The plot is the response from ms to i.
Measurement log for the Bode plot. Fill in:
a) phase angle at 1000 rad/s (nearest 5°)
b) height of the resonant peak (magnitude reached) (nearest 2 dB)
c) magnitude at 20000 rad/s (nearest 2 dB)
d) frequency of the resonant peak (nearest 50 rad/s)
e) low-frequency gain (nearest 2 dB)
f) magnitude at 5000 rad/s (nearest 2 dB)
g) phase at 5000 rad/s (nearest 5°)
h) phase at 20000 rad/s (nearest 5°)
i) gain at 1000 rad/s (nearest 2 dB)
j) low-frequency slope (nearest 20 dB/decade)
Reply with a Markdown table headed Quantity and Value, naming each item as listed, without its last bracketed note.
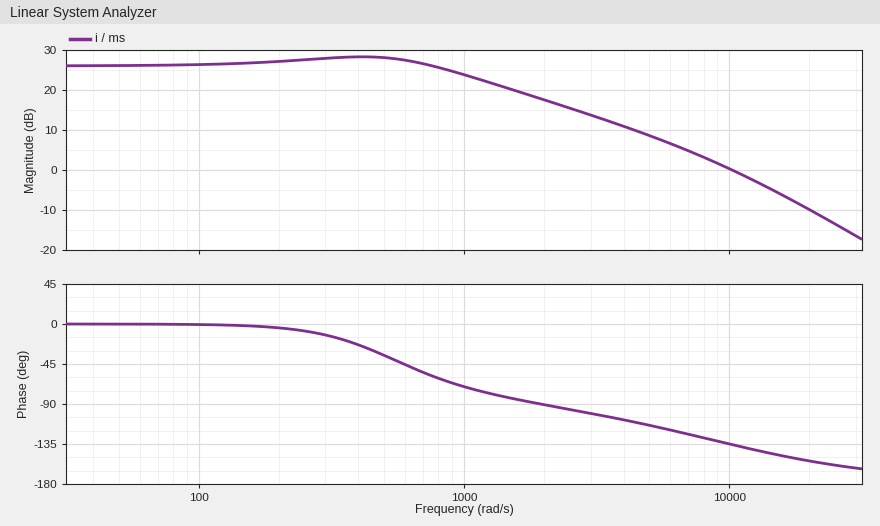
| Quantity | Value |
|---|---|
| phase angle at 1000 rad/s | -70° |
| height of the resonant peak (magnitude reached) | 28 dB |
| magnitude at 20000 rad/s | -10 dB |
| frequency of the resonant peak | 400 rad/s |
| low-frequency gain | 26 dB |
| magnitude at 5000 rad/s | 8 dB |
| phase at 5000 rad/s | -115° |
| phase at 20000 rad/s | -155° |
| gain at 1000 rad/s | 24 dB |
| low-frequency slope | 0 dB/decade |
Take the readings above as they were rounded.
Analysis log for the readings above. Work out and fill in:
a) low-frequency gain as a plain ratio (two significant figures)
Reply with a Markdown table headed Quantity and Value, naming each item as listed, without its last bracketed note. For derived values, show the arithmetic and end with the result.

| Quantity | Value |
|---|---|
| low-frequency gain as a plain ratio | 10^(26 / 20) = 20 |
